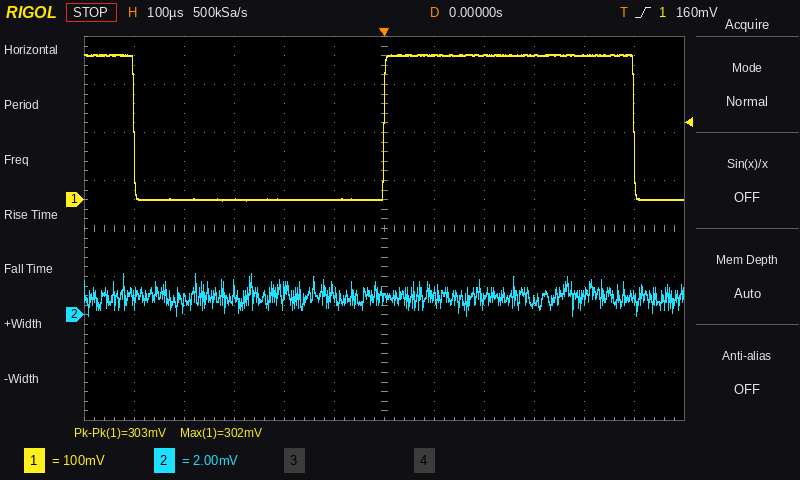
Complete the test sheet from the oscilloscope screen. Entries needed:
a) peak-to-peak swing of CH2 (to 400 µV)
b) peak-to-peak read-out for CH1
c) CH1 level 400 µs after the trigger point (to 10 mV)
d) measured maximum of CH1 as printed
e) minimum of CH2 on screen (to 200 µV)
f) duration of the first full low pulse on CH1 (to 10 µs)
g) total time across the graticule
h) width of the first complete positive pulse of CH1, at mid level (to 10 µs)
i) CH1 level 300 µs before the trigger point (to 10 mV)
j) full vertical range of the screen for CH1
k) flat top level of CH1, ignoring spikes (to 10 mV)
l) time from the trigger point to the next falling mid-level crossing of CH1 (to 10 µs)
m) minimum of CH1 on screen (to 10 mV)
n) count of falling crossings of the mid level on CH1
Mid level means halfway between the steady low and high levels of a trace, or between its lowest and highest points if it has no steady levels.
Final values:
1.6 mV
303 mV
300 mV
302 mV
0.0 mV
500 µs
1.2 ms
500 µs
0 mV
800 mV
300 mV
500 µs
0 mV
2
